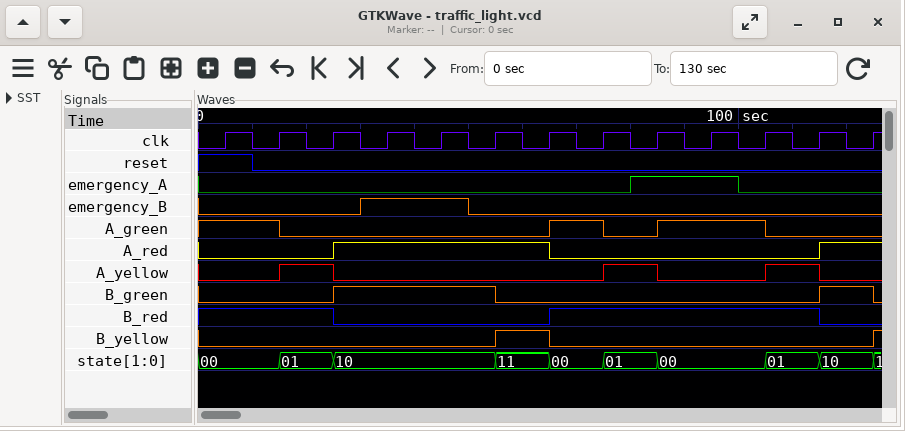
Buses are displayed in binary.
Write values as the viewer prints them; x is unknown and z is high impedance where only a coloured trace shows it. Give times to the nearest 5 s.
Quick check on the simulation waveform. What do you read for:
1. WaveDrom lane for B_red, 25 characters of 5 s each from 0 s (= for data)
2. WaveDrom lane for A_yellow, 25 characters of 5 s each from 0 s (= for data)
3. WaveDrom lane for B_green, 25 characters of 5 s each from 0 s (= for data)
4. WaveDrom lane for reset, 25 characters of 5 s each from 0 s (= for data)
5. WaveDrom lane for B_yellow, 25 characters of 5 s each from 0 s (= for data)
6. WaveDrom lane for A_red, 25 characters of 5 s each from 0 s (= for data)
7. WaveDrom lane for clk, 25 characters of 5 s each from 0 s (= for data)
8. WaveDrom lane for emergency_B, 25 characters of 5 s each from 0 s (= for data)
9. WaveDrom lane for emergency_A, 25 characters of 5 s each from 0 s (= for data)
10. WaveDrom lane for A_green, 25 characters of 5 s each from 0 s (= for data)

{name: 'B_red', wave: '1....0.......1.........0.'}
{name: 'A_yellow', wave: '0..1.0.........1.0...1.0.'}
{name: 'B_green', wave: '0....1.....0...........1.'}
{name: 'reset', wave: '1.0......................'}
{name: 'B_yellow', wave: '0..........1.0...........'}
{name: 'A_red', wave: '0....1.......0.........1.'}
{name: 'clk', wave: '0101010101010101010101010'}
{name: 'emergency_B', wave: '0.....1...0..............'}
{name: 'emergency_A', wave: '0...............1...0....'}
{name: 'A_green', wave: '1..0.........1.0.1...0...'}
